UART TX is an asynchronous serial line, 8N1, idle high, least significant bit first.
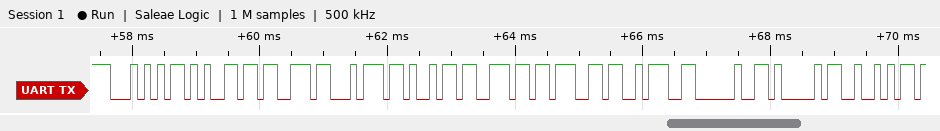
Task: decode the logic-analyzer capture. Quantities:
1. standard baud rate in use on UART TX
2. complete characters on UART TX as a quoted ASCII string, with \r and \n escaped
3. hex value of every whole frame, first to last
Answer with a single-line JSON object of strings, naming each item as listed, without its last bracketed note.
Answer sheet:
{"standard baud rate in use on UART TX": "9600 baud", "complete characters on UART TX as a quoted ASCII string, with \\r and \\n escaped": "\"Testing: AR\"", "hex value of every whole frame, first to last": "0x54 0x65 0x73 0x74 0x69 0x6E 0x67 0x3A 0x20 0x41 0x52"}
